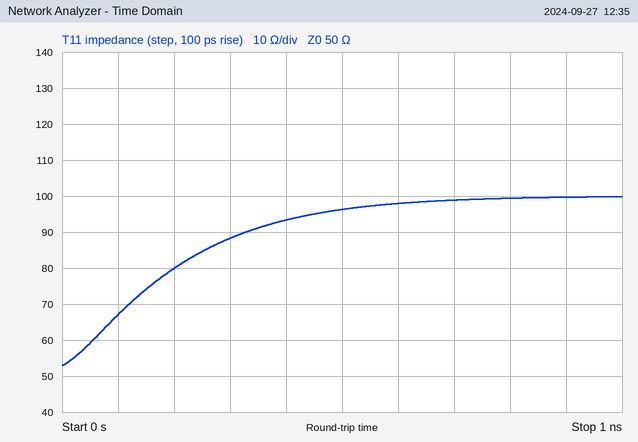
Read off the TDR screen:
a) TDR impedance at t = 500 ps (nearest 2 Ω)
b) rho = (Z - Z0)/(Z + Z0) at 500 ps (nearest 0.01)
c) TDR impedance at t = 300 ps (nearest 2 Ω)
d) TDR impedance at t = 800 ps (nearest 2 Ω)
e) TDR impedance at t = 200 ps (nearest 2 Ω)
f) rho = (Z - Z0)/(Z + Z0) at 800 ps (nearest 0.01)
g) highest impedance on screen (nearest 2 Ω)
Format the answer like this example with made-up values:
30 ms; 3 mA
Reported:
96 Ω; +0.32; 88 Ω; 100 Ω; 80 Ω; +0.33; 100 Ω
